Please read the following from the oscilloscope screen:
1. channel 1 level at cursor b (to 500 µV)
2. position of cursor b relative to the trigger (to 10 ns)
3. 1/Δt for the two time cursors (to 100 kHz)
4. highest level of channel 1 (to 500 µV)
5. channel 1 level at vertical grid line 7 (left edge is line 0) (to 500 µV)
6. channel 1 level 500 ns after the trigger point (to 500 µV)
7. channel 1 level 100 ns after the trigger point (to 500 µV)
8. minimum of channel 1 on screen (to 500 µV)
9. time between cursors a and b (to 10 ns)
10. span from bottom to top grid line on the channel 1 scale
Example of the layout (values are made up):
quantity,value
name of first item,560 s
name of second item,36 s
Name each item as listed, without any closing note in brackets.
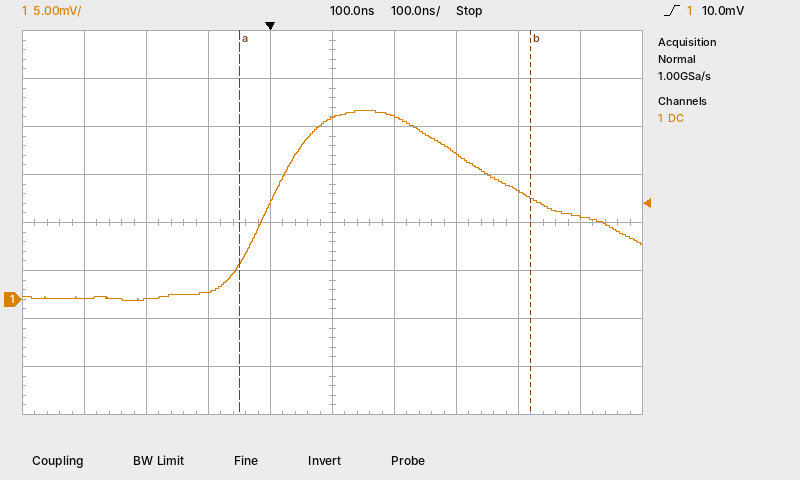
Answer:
quantity,value
channel 1 level at cursor b,10.5 mV
position of cursor b relative to the trigger,+420 ns
1/Δt for the two time cursors,2.1 MHz
highest level of channel 1,19.5 mV
channel 1 level at vertical grid line 7 (left edge is line 0),15.0 mV
channel 1 level 500 ns after the trigger point,8.5 mV
channel 1 level 100 ns after the trigger point,19.0 mV
minimum of channel 1 on screen,0.0 mV
time between cursors a and b,470 ns
span from bottom to top grid line on the channel 1 scale,40 mV
